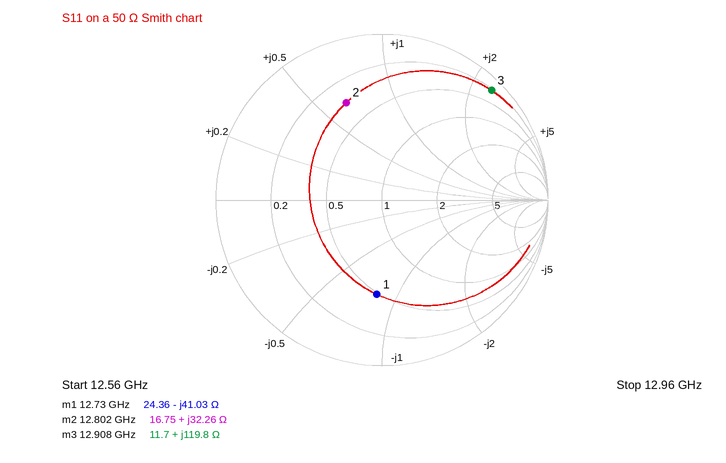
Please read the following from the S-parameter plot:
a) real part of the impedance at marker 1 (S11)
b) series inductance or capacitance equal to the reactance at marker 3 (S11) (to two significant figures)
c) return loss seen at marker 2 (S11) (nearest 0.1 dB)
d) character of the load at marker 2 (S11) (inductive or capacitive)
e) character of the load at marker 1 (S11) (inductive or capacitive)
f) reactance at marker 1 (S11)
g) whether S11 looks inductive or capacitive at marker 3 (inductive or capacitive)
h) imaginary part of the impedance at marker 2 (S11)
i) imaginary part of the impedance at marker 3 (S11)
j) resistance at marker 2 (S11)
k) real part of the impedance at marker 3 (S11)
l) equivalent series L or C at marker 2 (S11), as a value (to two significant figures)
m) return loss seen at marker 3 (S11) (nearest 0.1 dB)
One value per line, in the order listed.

24.36 Ω
1.5 nH
4.1 dB
inductive
capacitive
-41.03 Ω
inductive
+32.26 Ω
+119.8 Ω
16.75 Ω
11.7 Ω
400 pH
0.6 dB
